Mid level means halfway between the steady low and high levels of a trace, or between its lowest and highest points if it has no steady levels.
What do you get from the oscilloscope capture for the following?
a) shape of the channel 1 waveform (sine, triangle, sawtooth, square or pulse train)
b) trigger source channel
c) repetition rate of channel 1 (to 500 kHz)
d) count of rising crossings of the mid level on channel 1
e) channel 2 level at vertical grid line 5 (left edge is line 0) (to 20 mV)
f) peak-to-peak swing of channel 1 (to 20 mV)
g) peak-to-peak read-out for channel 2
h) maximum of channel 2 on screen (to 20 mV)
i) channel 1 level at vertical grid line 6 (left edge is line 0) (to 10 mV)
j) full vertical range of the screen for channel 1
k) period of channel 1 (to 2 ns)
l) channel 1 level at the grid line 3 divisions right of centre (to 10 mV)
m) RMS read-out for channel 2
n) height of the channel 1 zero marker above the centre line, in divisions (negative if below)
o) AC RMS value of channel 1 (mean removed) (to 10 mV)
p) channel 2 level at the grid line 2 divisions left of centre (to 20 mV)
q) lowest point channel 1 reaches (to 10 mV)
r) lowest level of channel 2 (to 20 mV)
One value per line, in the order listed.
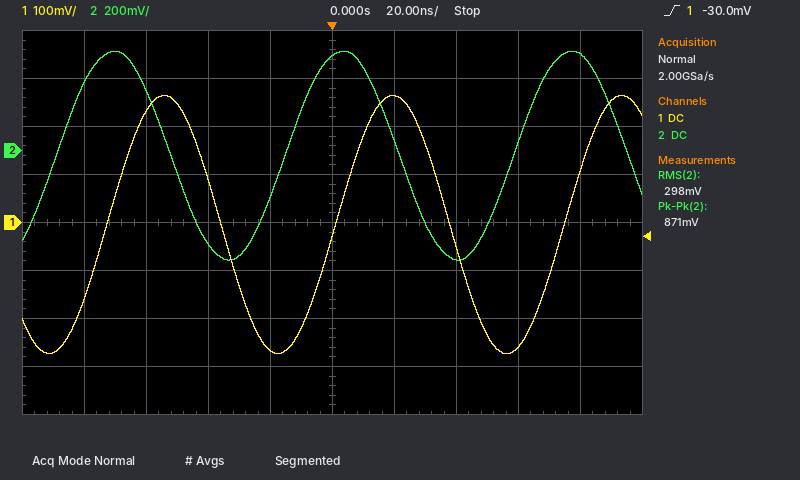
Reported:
sine
channel 1
13.5 MHz
3
400 mV
540 mV
871 mV
420 mV
260 mV
800 mV
74 ns
-260 mV
298 mV
0.0 div
190 mV
-380 mV
-270 mV
-460 mV
